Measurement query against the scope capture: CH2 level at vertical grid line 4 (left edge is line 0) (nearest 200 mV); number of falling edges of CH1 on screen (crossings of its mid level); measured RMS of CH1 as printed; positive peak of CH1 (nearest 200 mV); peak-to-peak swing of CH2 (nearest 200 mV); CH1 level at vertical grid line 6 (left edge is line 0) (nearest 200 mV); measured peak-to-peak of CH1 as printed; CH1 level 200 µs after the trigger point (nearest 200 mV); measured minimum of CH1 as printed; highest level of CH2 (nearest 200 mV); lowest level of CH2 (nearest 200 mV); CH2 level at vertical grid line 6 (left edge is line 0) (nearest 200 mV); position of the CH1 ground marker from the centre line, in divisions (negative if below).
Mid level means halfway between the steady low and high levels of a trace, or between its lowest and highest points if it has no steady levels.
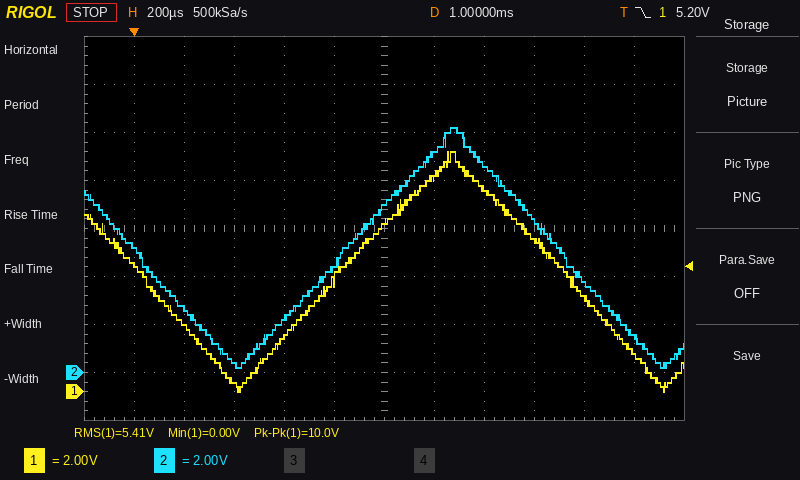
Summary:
2.2 V
2
5.41 V
10.0 V
10.0 V
7.0 V
10.0 V
2.8 V
0.00 V
10.2 V
200 mV
7.0 V
-3.4 div
